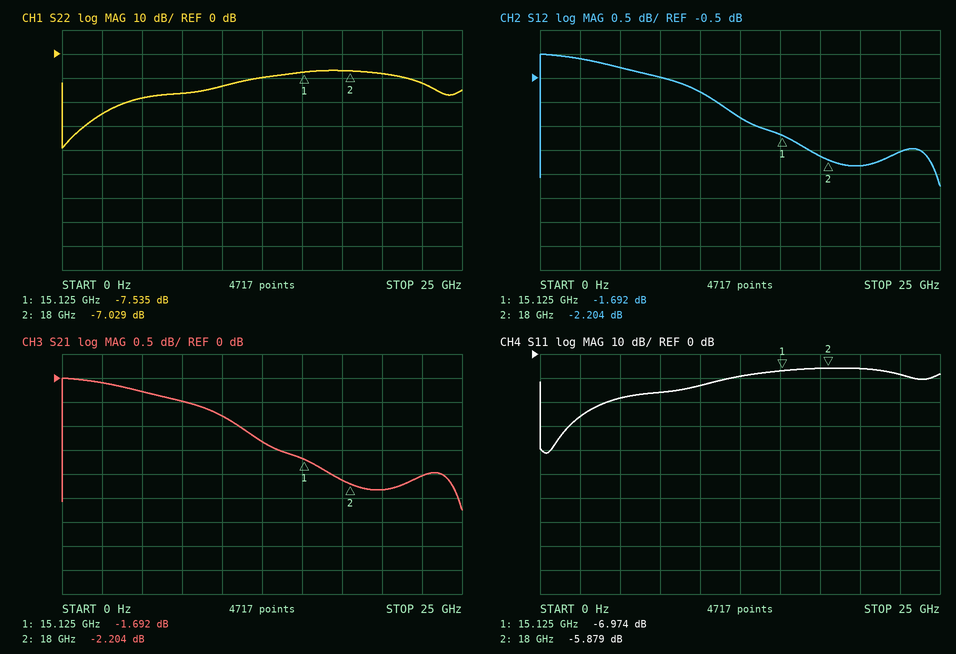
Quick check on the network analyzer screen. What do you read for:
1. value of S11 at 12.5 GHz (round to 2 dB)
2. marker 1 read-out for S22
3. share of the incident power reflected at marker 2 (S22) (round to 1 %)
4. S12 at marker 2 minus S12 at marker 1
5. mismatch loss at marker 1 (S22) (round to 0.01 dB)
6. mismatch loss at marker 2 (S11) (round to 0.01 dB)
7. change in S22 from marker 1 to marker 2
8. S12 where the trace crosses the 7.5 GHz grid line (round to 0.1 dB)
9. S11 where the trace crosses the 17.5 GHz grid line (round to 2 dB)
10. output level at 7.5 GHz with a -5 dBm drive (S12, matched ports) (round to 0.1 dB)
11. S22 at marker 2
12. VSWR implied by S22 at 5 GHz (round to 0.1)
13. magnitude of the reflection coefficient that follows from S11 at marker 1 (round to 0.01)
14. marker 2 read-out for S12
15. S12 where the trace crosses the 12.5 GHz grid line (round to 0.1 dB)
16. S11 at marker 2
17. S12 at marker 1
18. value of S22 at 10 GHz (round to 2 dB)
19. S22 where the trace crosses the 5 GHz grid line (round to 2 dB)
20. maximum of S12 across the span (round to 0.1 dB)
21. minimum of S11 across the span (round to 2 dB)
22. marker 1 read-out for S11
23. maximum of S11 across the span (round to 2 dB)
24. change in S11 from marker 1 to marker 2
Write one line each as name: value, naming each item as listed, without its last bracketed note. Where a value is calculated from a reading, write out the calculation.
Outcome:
value of S11 at 12.5 GHz: -10 dB
marker 1 read-out for S22: -7.535 dB
share of the incident power reflected at marker 2 (S22): 10^(-7.029/10) ≈ 20 %
S12 at marker 2 minus S12 at marker 1: -2.204 − (-1.692) = -0.512 dB
mismatch loss at marker 1 (S22): −10 log10(1 − 10^(-7.535/10)) ≈ 0.84 dB
mismatch loss at marker 2 (S11): −10 log10(1 − 10^(-5.879/10)) ≈ 1.30 dB
change in S22 from marker 1 to marker 2: -7.029 − (-7.535) = 0.506 dB
S12 where the trace crosses the 7.5 GHz grid line: -0.5 dB
S11 where the trace crosses the 17.5 GHz grid line: -6 dB
output level at 7.5 GHz with a -5 dBm drive (S12, matched ports): -5 dBm + (-0.5 dB) = -5.5 dBm
S22 at marker 2: -7.029 dB
VSWR implied by S22 at 5 GHz: |Γ| = 10^(-18/20) = 0.1259; VSWR = (1 + 0.1259)/(1 − 0.1259) ≈ 1.3
magnitude of the reflection coefficient that follows from S11 at marker 1: 10^(-6.974/20) ≈ 0.45
marker 2 read-out for S12: -2.204 dB
S12 where the trace crosses the 12.5 GHz grid line: -1.3 dB
S11 at marker 2: -5.879 dB
S12 at marker 1: -1.692 dB
value of S22 at 10 GHz: -14 dB
S22 where the trace crosses the 5 GHz grid line: -18 dB
maximum of S12 across the span: 0.0 dB
minimum of S11 across the span: -42 dB
marker 1 read-out for S11: -6.974 dB
maximum of S11 across the span: -6 dB
change in S11 from marker 1 to marker 2: -5.879 − (-6.974) = 1.095 dB
